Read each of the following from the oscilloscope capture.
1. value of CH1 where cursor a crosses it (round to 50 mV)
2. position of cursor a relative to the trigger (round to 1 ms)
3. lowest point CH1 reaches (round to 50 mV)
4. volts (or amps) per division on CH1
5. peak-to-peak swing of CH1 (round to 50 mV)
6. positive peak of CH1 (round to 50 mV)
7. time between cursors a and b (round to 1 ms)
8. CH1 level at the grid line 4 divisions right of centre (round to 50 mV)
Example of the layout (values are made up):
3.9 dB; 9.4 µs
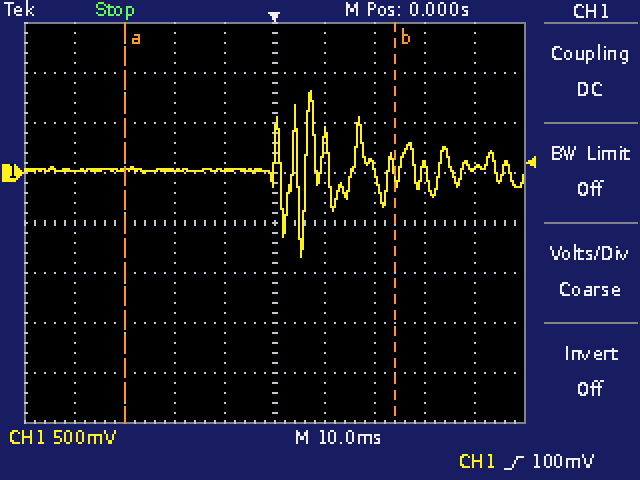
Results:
50 mV; -30 ms; -850 mV; 500 mV; 1.65 V; 800 mV; 54 ms; 50 mV
